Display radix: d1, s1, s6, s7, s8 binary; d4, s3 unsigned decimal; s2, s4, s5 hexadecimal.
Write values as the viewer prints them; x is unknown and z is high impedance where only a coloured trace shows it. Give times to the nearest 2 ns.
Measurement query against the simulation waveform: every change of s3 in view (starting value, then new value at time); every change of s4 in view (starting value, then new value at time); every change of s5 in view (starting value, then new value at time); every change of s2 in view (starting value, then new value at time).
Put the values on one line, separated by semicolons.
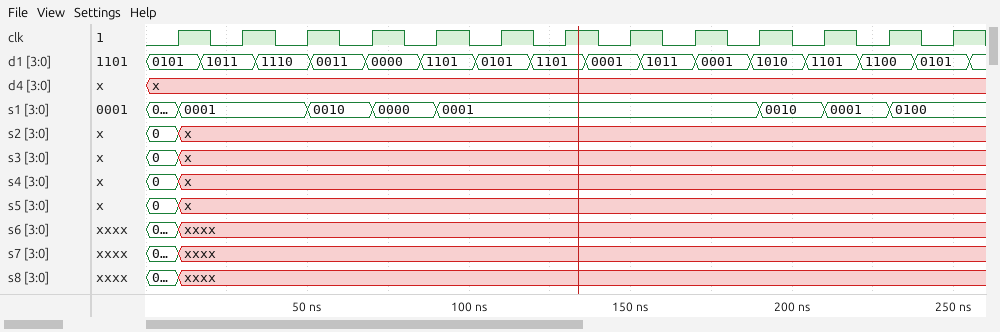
0, x at 10 ns; 0, x at 10 ns; 0, x at 10 ns; 0, x at 10 ns
